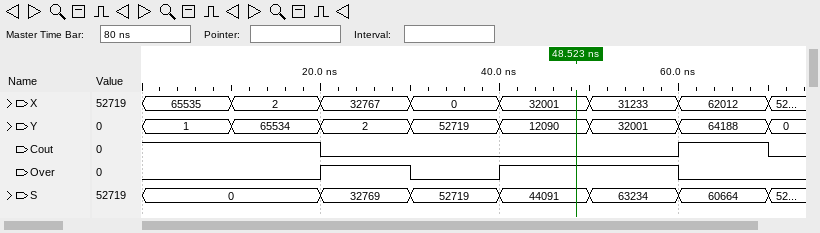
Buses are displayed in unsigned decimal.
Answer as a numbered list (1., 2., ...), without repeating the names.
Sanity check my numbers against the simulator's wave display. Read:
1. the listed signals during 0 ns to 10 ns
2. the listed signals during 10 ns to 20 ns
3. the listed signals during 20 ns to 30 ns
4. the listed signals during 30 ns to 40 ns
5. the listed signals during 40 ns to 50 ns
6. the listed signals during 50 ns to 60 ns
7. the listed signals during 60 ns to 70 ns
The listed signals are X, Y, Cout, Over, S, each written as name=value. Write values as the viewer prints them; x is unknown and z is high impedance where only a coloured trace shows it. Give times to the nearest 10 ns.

1. X=65535, Y=1, Cout=1, Over=0, S=0
2. X=2, Y=65534, Cout=1, Over=0, S=0
3. X=32767, Y=2, Cout=0, Over=1, S=32769
4. X=0, Y=52719, Cout=0, Over=0, S=52719
5. X=32001, Y=12090, Cout=0, Over=1, S=44091
6. X=31233, Y=32001, Cout=0, Over=1, S=63234
7. X=62012, Y=64188, Cout=1, Over=0, S=60664
